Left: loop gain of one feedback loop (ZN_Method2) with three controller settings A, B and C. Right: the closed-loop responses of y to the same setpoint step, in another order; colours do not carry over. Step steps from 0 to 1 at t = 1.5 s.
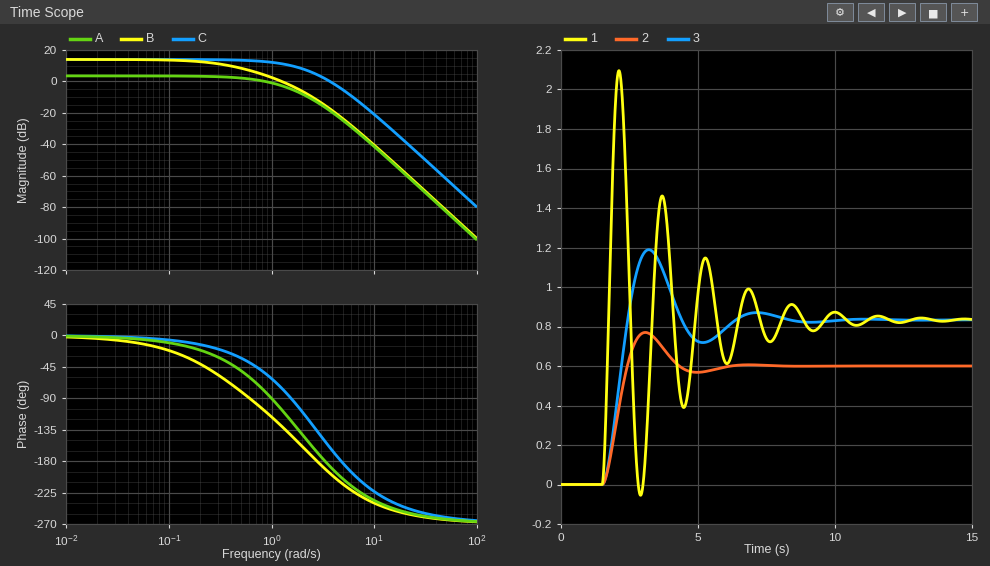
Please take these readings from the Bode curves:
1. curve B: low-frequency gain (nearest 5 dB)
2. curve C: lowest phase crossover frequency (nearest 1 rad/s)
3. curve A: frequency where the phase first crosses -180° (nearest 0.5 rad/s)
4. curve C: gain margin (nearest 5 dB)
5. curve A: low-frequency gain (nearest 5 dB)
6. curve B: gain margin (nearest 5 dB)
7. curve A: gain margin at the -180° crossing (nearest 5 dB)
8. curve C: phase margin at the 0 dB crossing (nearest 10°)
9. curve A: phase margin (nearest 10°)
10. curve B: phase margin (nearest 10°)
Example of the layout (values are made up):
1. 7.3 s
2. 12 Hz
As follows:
1. 15 dB
2. 5 rad/s
3. 3.5 rad/s
4. 5 dB
5. 5 dB
6. 10 dB
7. 15 dB
8. 20°
9. 100°
10. 50°
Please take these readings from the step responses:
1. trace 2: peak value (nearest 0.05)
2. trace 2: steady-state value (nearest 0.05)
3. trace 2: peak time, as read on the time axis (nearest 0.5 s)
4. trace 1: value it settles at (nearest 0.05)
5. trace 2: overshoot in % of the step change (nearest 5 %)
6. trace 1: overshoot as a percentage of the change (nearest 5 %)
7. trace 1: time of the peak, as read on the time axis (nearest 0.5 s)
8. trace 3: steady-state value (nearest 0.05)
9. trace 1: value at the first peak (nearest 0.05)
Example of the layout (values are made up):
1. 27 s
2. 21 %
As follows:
1. 0.75
2. 0.60
3. 3.0 s
4. 0.85
5. 30 %
6. 150 %
7. 2.0 s
8. 0.85
9. 2.10
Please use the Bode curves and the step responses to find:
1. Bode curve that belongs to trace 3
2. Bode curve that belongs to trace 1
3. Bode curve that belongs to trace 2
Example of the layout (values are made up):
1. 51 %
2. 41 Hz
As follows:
1. B
2. C
3. A
